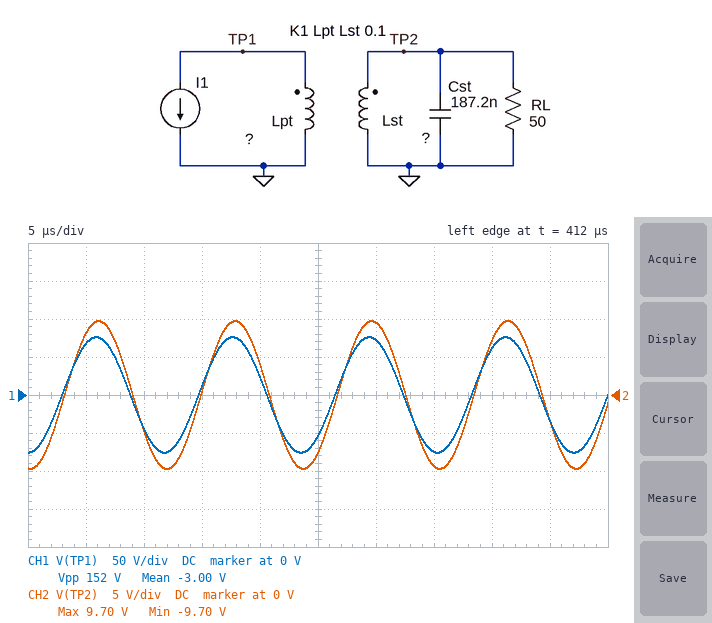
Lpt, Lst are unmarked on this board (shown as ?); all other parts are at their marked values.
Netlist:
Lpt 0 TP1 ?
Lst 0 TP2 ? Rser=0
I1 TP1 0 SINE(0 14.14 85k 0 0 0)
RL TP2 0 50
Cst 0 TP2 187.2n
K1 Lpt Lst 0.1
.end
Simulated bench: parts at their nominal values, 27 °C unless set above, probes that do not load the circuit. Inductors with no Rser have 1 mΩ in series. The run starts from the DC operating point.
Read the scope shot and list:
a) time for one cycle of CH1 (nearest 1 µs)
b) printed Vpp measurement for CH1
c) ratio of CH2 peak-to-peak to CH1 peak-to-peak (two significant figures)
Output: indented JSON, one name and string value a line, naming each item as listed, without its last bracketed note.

{
  "time for one cycle of CH1": "12 µs",
  "printed Vpp measurement for CH1": "152 V",
  "ratio of CH2 peak-to-peak to CH1 peak-to-peak": "0.13"
}
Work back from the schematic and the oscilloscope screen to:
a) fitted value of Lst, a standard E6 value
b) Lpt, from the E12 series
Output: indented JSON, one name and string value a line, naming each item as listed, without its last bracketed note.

{
  "fitted value of Lst, a standard E6 value": "6.8 µH",
  "Lpt, from the E12 series": "10 µH"
}
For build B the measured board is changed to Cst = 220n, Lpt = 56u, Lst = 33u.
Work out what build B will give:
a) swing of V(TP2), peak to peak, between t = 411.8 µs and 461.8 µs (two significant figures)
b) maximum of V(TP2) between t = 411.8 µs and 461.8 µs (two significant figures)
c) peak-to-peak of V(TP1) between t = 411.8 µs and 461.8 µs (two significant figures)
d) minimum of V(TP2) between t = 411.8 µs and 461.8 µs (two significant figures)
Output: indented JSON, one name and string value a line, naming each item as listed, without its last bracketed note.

{
  "swing of V(TP2), peak to peak, between t = 411.8 µs and 461.8 µs": "58 V",
  "maximum of V(TP2) between t = 411.8 µs and 461.8 µs": "29 V",
  "peak-to-peak of V(TP1) between t = 411.8 µs and 461.8 µs": "830 V",
  "minimum of V(TP2) between t = 411.8 µs and 461.8 µs": "-29 V"
}
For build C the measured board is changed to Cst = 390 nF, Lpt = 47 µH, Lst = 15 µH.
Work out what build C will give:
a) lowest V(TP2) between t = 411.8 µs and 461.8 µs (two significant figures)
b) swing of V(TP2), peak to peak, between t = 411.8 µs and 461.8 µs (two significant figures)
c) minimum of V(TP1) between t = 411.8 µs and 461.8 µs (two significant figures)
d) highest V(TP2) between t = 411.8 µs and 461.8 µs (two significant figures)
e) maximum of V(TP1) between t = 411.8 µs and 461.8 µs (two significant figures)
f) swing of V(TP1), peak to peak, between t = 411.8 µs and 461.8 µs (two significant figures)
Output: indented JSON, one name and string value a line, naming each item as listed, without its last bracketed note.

{
  "lowest V(TP2) between t = 411.8 µs and 461.8 µs": "-29 V",
  "swing of V(TP2), peak to peak, between t = 411.8 µs and 461.8 µs": "58 V",
  "minimum of V(TP1) between t = 411.8 µs and 461.8 µs": "-350 V",
  "highest V(TP2) between t = 411.8 µs and 461.8 µs": "29 V",
  "maximum of V(TP1) between t = 411.8 µs and 461.8 µs": "350 V",
  "swing of V(TP1), peak to peak, between t = 411.8 µs and 461.8 µs": "690 V"
}
